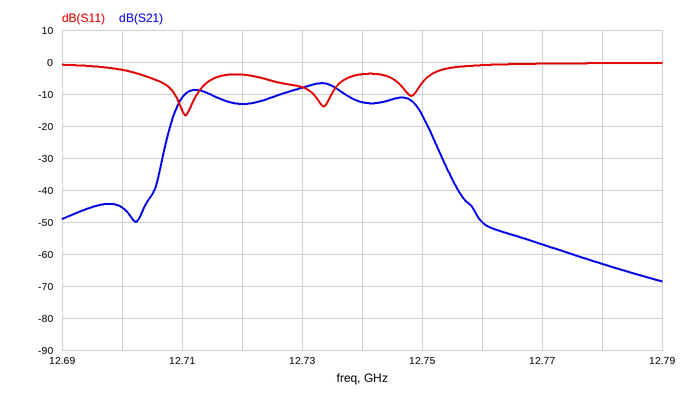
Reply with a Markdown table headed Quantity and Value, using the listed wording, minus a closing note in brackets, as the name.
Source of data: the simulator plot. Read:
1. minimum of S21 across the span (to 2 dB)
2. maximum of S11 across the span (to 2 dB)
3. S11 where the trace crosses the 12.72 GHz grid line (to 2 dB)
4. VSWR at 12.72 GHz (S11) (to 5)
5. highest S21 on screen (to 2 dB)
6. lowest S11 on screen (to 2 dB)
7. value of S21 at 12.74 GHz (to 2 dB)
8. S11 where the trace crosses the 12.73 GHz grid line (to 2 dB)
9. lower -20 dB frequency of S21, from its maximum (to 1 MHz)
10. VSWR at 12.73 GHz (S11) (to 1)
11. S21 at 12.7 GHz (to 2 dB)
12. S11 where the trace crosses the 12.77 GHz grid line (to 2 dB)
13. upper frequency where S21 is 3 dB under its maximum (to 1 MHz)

| Quantity | Value |
|---|---|
| minimum of S21 across the span | -68 dB |
| maximum of S11 across the span | 0 dB |
| S11 where the trace crosses the 12.72 GHz grid line | -4 dB |
| VSWR at 12.72 GHz (S11) | 5 |
| highest S21 on screen | -6 dB |
| lowest S11 on screen | -16 dB |
| value of S21 at 12.74 GHz | -12 dB |
| S11 where the trace crosses the 12.73 GHz grid line | -8 dB |
| lower -20 dB frequency of S21, from its maximum | 12.707 GHz |
| VSWR at 12.73 GHz (S11) | 2 |
| S21 at 12.7 GHz | -46 dB |
| S11 where the trace crosses the 12.77 GHz grid line | 0 dB |
| upper frequency where S21 is 3 dB under its maximum | 12.737 GHz |
